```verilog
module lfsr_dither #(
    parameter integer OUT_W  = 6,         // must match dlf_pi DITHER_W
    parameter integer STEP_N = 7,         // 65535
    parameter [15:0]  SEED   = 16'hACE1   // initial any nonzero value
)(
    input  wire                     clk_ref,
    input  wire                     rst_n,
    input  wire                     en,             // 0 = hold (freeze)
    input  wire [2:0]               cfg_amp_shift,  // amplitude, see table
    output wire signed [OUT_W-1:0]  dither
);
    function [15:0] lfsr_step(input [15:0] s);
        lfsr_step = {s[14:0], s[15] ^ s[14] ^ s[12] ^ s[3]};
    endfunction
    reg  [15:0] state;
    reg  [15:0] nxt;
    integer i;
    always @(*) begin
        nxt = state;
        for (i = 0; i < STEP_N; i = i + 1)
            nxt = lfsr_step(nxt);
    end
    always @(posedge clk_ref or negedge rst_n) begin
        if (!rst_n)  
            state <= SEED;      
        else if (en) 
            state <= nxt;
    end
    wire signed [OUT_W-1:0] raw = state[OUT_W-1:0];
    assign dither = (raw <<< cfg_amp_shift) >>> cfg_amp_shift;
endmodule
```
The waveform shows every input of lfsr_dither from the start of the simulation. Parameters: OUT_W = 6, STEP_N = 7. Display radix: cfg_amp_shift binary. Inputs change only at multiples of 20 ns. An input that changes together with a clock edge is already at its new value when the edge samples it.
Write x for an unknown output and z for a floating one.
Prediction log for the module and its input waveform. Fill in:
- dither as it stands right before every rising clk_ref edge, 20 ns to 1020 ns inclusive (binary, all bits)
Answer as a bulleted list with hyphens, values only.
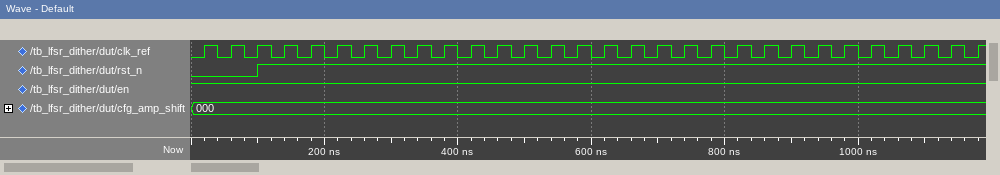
- 100001, 100001, 100001, 000101, 100001, 010100, 011010, 100101, 010110, 100011, 011111, 100000, 100101, 100110, 100110, 110100, 000110, 001111, 110001, 010110, 010010, 100101, 110111, 011001, 100110, 101011
